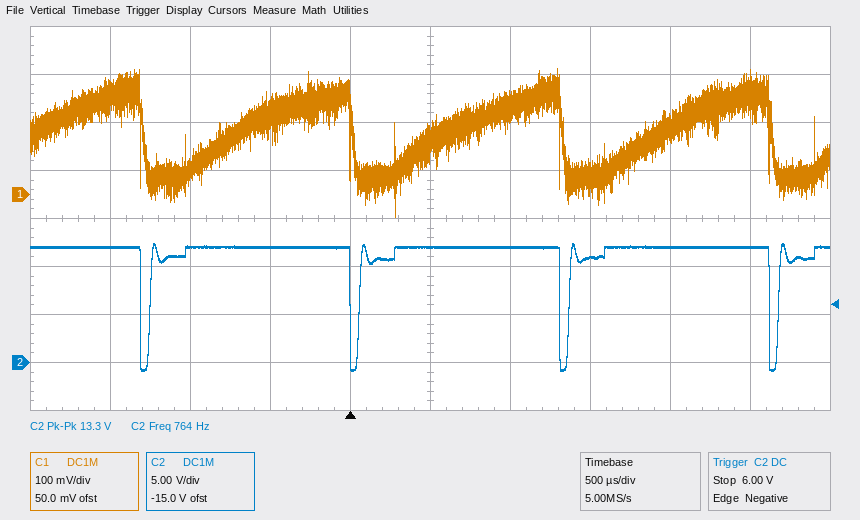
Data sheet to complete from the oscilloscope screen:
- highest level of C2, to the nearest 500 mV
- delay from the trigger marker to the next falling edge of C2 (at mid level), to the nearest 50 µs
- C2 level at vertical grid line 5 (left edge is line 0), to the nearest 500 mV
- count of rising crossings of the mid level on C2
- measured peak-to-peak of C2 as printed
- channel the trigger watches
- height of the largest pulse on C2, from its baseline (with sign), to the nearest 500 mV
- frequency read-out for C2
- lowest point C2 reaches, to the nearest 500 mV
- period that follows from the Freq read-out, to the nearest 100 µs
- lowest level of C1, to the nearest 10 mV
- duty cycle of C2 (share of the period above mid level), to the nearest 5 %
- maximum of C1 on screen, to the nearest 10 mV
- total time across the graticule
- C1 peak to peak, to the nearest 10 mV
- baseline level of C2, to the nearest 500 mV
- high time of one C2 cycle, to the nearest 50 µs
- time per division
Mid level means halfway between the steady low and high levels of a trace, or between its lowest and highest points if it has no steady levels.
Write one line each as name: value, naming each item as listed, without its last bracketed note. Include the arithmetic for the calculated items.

highest level of C2, to the nearest 500 mV: 12.5 V
delay from the trigger marker to the next falling edge of C2 (at mid level), to the nearest 50 µs: 1.30 ms
C2 level at vertical grid line 5 (left edge is line 0), to the nearest 500 mV: 12.0 V
count of rising crossings of the mid level on C2: 4
measured peak-to-peak of C2 as printed: 13.3 V
channel the trigger watches: C2
height of the largest pulse on C2, from its baseline (with sign), to the nearest 500 mV: -1.0 V − (12.0 V) = -13.0 V
frequency read-out for C2: 764 Hz
lowest point C2 reaches, to the nearest 500 mV: -1.0 V
period that follows from the Freq read-out, to the nearest 100 µs: 1 / 764 Hz ≈ 1.3 ms
lowest level of C1, to the nearest 10 mV: -50 mV
duty cycle of C2 (share of the period above mid level), to the nearest 5 %: 95 %
maximum of C1 on screen, to the nearest 10 mV: 260 mV
total time across the graticule: 5 ms
C1 peak to peak, to the nearest 10 mV: 260 mV − (-50 mV) = 310 mV
baseline level of C2, to the nearest 500 mV: 12.0 V
high time of one C2 cycle, to the nearest 50 µs: 1.25 ms
time per division: 500 µs
